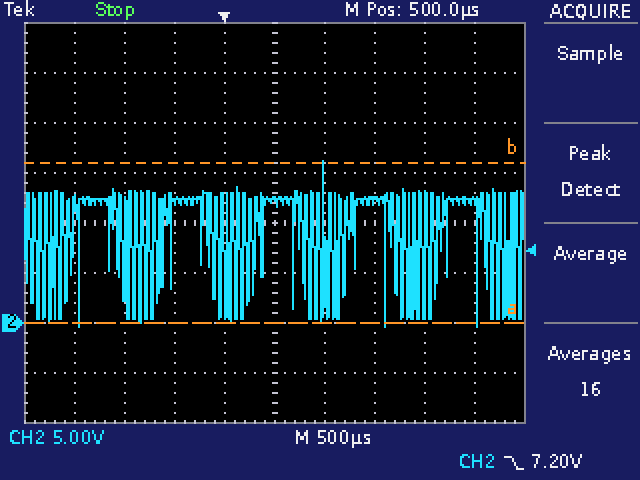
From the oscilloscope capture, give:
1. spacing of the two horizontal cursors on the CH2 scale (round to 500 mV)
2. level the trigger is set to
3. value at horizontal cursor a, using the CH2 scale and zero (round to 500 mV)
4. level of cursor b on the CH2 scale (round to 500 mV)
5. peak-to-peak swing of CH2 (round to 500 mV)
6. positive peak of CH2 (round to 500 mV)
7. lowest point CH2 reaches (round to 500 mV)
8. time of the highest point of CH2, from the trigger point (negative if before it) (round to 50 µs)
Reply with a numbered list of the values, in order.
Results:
1. 16.0 V
2. 7.20 V
3. 0.0 V
4. 16.0 V
5. 16.5 V
6. 16.0 V
7. -500 mV
8. +1.00 ms
